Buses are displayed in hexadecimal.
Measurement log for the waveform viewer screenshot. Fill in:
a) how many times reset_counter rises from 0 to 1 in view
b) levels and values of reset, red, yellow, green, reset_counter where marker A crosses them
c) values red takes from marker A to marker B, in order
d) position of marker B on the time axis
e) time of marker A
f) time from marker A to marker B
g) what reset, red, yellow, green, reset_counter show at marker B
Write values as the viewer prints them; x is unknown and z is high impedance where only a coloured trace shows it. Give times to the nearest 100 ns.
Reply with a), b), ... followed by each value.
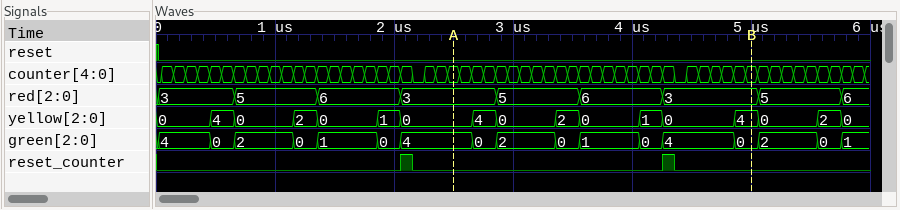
a) 2
b) reset=0, red=3, yellow=0, green=4, reset_counter=0
c) 3, 5, 6, 3
d) 5000 ns
e) 2500 ns
f) 2500 ns
g) reset=0, red=3, yellow=4, green=0, reset_counter=0
